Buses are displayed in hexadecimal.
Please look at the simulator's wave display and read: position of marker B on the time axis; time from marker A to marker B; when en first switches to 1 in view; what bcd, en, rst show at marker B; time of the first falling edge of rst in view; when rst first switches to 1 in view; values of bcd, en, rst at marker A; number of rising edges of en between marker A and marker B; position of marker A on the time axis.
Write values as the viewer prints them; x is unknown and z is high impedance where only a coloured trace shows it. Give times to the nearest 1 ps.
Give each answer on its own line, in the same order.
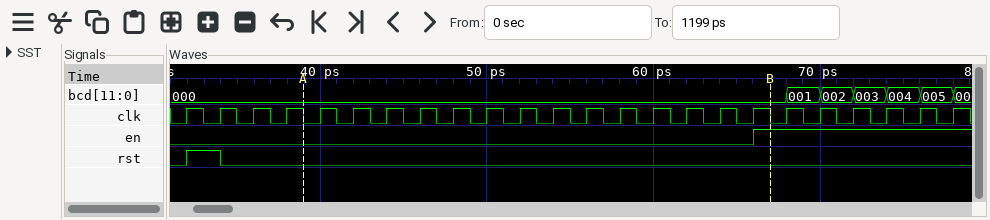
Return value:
67 ps
28 ps
66 ps
bcd=000, en=1, rst=0
34 ps
32 ps
bcd=000, en=0, rst=0
1
39 ps
